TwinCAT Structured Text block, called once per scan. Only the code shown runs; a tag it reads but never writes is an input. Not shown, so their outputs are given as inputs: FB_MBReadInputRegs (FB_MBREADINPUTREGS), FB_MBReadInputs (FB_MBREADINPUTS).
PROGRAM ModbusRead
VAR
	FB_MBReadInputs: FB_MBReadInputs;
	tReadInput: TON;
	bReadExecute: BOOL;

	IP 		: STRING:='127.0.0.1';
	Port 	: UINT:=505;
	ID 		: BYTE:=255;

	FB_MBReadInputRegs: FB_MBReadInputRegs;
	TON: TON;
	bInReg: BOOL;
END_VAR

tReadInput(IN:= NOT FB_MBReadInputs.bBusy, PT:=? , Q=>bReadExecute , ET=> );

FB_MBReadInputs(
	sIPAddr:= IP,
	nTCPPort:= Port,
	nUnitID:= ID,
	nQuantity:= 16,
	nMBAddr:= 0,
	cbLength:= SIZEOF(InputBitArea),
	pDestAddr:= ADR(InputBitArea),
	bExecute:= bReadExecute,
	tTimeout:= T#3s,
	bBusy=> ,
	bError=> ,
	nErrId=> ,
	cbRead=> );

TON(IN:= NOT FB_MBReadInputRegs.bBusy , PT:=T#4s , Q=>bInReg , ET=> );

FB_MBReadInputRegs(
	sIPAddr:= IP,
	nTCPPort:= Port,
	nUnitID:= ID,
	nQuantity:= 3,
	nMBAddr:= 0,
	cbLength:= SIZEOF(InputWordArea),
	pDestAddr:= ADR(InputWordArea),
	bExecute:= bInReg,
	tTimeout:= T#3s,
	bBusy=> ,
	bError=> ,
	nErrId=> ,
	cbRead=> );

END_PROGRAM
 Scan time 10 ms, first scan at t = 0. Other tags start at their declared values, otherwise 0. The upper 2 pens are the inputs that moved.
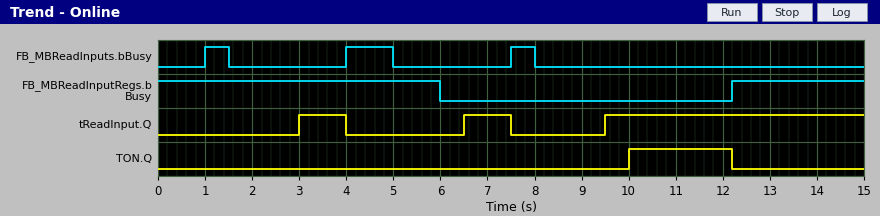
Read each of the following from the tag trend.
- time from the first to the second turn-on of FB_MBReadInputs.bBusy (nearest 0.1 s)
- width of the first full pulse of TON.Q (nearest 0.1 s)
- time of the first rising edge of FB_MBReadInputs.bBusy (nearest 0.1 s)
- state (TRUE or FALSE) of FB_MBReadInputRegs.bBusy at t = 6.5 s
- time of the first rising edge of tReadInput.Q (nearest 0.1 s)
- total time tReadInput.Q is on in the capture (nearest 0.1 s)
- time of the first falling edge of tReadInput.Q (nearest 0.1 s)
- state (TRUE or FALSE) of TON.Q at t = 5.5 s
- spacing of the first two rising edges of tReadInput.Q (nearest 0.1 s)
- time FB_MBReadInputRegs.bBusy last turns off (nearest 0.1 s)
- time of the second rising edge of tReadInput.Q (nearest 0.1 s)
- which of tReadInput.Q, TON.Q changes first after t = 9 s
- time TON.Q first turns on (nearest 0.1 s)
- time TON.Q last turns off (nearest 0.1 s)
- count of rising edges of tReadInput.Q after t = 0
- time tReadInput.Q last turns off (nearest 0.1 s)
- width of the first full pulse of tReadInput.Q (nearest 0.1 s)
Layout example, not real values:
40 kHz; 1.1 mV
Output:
3.0 s; 2.2 s; 1.0 s; FALSE; 3.0 s; 7.5 s; 4.0 s; FALSE; 3.5 s; 6.0 s; 6.5 s; tReadInput.Q; 10.0 s; 12.2 s; 3; 7.5 s; 1.0 s
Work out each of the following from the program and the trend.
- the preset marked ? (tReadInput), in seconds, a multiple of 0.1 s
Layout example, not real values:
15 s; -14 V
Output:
1.5 s
